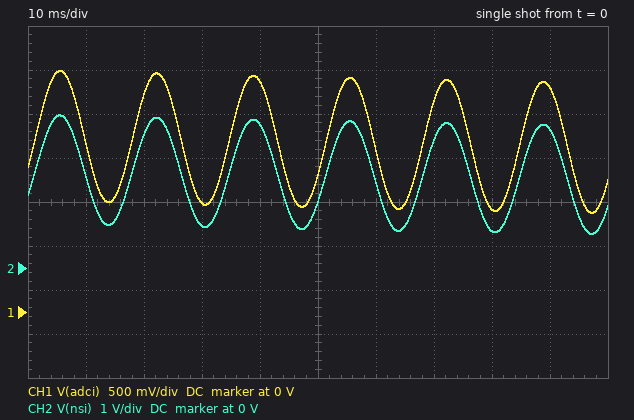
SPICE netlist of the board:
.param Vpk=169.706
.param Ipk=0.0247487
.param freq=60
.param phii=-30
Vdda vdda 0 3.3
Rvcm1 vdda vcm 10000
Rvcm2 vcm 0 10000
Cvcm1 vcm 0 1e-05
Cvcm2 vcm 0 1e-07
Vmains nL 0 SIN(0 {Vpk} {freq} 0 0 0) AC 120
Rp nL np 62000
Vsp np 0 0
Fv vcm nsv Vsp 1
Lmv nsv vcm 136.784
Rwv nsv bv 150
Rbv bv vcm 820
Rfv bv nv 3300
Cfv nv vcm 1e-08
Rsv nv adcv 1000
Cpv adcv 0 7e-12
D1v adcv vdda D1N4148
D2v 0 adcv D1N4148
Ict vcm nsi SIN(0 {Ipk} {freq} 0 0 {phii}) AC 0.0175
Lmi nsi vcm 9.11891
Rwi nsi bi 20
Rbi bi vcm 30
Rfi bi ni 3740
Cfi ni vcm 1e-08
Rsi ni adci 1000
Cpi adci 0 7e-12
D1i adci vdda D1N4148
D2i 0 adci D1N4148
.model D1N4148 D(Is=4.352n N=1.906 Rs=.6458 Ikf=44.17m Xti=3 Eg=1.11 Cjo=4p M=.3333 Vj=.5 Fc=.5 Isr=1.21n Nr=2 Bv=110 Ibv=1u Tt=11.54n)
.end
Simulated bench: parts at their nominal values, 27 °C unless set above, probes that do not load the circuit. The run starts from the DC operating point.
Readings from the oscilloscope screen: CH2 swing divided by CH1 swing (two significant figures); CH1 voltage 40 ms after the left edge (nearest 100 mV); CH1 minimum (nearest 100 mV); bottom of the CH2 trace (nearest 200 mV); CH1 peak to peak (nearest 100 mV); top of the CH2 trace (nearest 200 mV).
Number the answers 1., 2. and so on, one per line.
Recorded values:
1. 1.7
2. 2.6 V
3. 1.1 V
4. 800 mV
5. 1.6 V
6. 3.4 V
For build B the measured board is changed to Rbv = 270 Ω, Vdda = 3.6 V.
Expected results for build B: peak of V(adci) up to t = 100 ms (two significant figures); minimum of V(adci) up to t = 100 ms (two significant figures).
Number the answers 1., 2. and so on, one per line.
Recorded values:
1. 2.9 V
2. 1.3 V
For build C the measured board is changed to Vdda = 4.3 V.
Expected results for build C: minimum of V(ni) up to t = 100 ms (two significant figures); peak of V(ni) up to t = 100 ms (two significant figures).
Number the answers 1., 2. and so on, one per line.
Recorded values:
1. 1.6 V
2. 3.2 V
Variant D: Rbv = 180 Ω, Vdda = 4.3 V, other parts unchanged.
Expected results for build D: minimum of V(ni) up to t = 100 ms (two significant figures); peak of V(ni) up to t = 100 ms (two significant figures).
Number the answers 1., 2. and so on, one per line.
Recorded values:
1. 1.6 V
2. 3.2 V
